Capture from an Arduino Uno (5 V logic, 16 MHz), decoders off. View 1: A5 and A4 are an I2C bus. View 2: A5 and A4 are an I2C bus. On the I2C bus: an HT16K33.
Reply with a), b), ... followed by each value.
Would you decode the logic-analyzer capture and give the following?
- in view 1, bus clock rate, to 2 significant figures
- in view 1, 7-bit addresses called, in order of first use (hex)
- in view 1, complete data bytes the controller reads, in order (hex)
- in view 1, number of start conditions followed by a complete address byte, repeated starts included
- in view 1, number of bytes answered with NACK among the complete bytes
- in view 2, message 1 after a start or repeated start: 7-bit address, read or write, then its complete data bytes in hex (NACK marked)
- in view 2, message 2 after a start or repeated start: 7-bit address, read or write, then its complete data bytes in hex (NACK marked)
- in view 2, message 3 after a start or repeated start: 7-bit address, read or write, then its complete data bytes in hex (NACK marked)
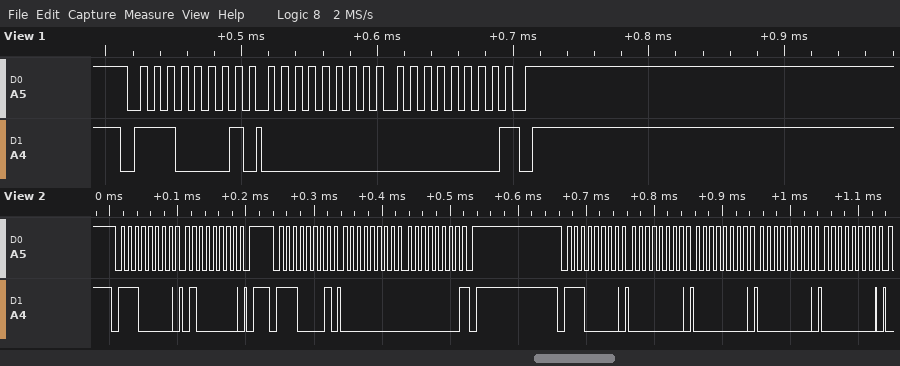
a) 100 kHz
b) 0x70
c) 00 00
d) 1
e) 1
f) 0x70 write: 40
g) 0x70 read: 00 00 NACK
h) 0x70 write: 00 00 00 00
